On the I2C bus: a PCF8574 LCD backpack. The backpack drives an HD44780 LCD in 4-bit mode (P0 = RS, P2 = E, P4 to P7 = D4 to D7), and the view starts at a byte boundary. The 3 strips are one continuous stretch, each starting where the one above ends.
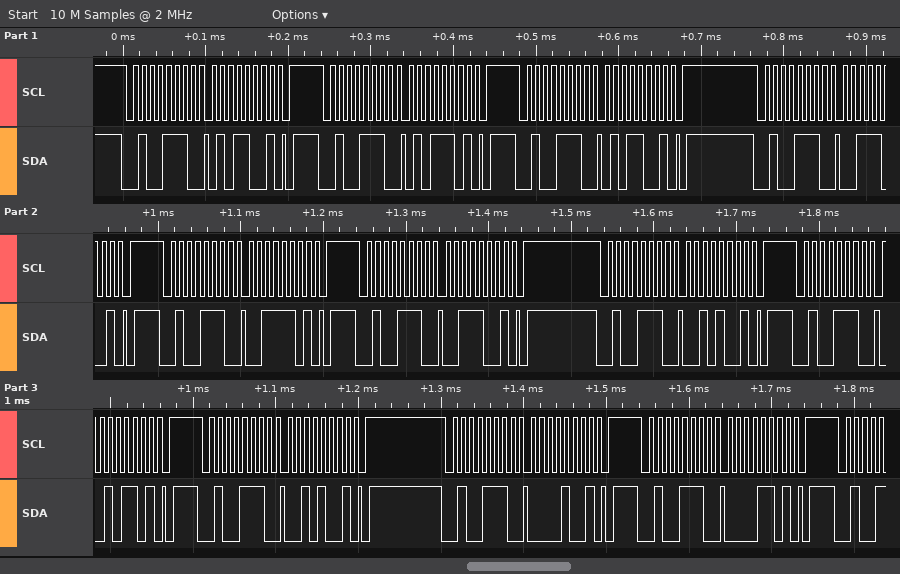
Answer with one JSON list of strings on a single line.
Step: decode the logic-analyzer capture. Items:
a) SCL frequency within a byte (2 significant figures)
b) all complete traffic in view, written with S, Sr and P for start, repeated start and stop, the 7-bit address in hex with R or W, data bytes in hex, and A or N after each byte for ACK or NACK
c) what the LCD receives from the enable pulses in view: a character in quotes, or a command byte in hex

["100 kHz", "S 27W A 59 A P S 27W A 5D A P S 27W A 59 A P S 27W A 39 A P S 27W A 3D A P S 27W A 39 A P S 27W A 29 A P S 27W A 2D A P S 27W A 29 A P S 27W A 09 A P S 27W A 0D A P", "'S'"]
